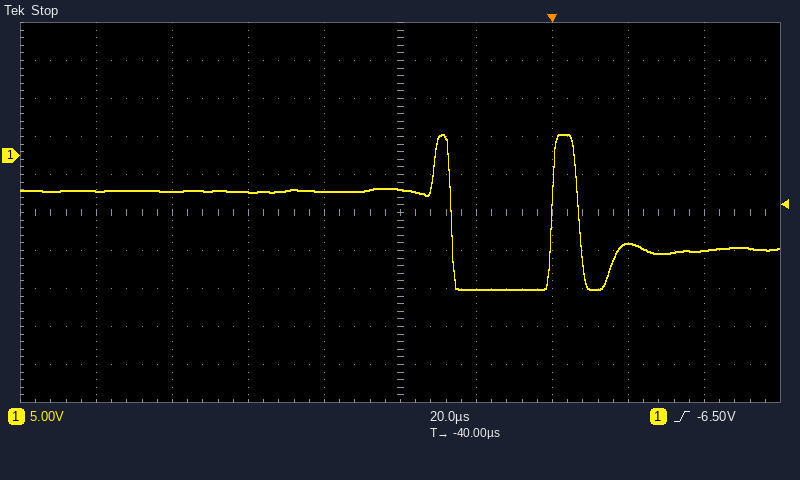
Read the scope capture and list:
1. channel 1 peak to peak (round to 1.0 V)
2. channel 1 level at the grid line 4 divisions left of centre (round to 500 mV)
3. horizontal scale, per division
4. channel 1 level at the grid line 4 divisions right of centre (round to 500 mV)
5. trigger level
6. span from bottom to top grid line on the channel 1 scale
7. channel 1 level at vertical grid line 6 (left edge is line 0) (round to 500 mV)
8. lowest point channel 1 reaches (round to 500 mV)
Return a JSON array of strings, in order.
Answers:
["20.0 V", "-4.5 V", "20 µs", "-12.5 V", "-6.50 V", "50 V", "-17.5 V", "-17.5 V"]
